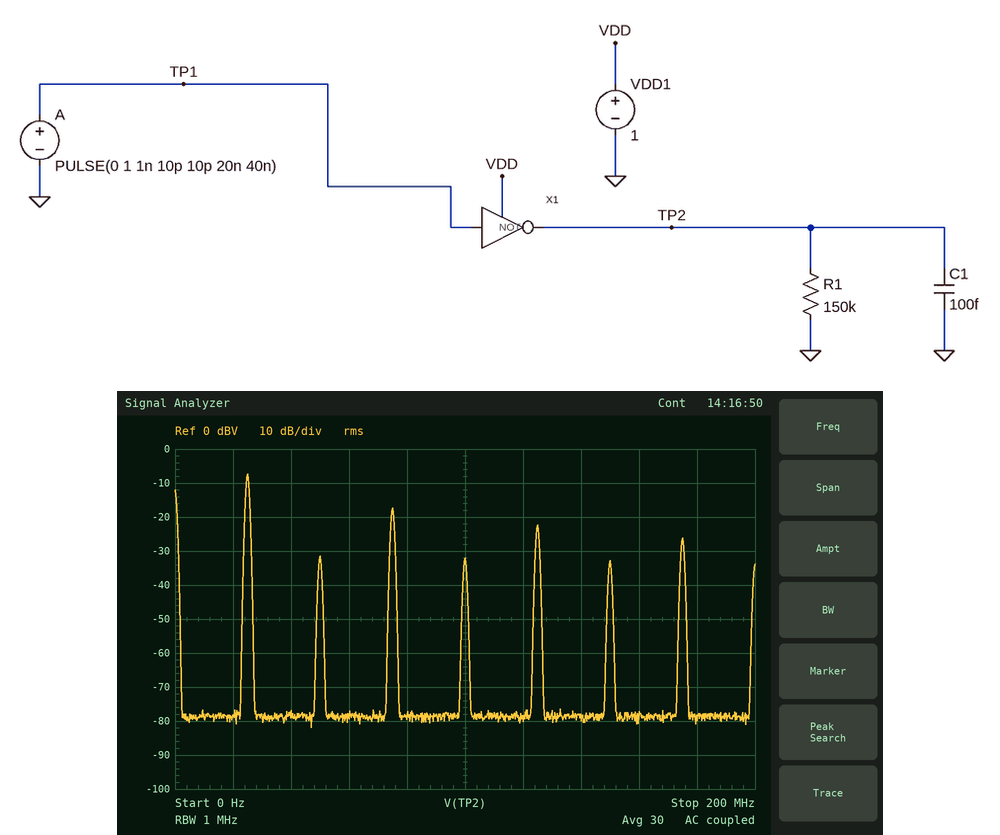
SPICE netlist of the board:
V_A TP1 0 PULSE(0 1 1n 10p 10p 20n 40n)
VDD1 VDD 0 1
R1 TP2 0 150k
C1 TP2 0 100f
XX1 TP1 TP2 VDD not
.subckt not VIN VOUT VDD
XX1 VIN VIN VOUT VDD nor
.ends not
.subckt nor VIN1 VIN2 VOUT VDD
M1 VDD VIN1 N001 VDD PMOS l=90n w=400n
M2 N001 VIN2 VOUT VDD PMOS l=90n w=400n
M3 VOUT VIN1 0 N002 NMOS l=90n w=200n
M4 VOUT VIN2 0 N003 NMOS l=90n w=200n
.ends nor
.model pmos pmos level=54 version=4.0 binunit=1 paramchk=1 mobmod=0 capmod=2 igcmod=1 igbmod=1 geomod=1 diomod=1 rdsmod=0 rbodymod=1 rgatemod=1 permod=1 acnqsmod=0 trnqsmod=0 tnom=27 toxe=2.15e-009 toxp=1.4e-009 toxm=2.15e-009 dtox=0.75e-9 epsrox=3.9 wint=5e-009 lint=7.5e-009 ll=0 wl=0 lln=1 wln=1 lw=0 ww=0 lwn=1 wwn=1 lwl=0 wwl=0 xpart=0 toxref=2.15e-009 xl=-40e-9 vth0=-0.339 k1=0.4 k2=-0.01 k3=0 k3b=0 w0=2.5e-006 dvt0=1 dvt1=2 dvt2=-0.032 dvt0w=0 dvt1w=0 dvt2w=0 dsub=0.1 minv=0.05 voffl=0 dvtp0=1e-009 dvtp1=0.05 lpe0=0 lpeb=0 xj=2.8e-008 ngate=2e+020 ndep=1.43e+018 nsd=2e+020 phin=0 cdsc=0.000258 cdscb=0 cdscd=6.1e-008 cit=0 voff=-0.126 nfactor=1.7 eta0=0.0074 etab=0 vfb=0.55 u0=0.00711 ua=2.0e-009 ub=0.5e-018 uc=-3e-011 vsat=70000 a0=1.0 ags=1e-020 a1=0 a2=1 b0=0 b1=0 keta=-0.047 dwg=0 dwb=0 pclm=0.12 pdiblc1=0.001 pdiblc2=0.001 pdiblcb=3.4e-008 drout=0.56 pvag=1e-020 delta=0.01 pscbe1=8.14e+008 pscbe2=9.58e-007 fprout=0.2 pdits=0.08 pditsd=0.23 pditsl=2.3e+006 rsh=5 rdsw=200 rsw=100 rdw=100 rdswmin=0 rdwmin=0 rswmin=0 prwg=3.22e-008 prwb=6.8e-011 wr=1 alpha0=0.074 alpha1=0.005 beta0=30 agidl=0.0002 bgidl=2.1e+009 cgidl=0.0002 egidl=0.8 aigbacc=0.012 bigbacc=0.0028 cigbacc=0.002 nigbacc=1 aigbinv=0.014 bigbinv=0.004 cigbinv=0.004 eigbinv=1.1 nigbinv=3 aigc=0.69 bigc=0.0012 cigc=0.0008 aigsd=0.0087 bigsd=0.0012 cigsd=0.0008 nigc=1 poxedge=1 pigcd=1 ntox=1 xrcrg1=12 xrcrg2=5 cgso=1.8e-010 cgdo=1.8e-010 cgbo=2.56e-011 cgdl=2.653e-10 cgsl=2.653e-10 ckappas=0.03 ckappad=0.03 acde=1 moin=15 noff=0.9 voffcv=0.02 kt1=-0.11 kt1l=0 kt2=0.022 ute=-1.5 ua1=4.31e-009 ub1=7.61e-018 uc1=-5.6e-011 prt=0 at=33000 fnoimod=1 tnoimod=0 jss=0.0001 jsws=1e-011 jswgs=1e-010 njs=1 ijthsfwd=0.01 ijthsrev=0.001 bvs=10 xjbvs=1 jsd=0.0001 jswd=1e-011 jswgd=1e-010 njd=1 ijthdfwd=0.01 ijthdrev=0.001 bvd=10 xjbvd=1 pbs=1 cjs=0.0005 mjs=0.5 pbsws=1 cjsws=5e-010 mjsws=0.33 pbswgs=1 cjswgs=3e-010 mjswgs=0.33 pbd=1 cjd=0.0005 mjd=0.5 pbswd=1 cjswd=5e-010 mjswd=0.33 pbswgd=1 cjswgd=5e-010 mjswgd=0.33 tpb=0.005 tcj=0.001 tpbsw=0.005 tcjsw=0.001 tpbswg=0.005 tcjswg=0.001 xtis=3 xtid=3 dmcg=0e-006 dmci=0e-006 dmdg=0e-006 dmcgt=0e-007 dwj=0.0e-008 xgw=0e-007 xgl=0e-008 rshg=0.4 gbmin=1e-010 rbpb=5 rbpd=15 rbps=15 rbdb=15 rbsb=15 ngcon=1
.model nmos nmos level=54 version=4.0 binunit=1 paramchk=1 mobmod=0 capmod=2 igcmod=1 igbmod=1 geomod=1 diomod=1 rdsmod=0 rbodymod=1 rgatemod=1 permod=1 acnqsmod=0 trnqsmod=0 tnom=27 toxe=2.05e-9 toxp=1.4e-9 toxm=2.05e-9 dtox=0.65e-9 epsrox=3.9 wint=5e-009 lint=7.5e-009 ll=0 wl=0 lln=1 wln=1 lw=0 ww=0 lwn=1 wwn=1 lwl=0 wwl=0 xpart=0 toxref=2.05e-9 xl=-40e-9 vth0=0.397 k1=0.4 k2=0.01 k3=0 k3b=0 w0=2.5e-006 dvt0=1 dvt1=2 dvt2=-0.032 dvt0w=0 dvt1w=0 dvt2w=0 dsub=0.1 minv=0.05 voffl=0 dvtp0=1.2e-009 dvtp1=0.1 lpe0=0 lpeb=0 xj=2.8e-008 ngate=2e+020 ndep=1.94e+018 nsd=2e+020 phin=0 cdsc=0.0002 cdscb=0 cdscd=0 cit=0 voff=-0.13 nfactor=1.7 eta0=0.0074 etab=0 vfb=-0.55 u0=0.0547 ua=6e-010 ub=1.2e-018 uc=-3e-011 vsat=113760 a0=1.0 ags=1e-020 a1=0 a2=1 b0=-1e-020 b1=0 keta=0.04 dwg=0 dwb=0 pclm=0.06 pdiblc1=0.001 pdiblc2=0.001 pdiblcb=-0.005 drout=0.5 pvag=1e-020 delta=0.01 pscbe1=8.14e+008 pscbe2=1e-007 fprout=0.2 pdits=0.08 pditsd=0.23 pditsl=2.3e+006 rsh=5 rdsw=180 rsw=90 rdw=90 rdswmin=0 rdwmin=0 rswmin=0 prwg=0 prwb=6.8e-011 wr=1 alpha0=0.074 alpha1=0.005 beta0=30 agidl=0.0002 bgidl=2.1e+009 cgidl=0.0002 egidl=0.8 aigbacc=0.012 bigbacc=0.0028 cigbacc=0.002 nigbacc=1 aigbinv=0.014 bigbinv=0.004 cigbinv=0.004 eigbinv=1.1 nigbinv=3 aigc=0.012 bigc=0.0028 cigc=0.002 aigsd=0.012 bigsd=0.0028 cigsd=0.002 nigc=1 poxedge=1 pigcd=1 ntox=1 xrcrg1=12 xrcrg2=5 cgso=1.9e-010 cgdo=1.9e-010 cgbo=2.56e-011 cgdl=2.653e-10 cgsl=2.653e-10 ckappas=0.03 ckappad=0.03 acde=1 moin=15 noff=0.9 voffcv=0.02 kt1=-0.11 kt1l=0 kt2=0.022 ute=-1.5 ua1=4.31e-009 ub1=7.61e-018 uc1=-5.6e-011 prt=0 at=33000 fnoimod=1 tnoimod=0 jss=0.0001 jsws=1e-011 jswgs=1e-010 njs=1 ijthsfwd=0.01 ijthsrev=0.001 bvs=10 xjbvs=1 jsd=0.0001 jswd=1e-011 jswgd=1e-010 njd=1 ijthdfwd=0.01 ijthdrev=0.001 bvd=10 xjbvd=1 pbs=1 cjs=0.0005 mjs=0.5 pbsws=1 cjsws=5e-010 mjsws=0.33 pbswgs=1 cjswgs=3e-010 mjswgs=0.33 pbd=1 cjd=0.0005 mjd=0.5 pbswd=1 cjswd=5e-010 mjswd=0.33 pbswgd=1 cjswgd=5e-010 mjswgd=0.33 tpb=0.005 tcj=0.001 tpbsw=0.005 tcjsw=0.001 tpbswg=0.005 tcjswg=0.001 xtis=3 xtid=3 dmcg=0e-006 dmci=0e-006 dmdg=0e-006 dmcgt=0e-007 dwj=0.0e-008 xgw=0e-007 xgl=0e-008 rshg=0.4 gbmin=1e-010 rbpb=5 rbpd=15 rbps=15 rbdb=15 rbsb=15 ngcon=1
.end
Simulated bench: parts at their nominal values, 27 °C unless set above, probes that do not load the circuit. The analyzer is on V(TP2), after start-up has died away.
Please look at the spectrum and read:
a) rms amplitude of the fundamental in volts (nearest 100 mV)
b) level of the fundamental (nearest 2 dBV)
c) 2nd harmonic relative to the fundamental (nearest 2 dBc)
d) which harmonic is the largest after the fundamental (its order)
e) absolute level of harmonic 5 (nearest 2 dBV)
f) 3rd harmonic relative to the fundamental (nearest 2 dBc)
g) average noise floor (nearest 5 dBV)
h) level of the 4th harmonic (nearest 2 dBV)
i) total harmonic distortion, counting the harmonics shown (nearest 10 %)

400 mV
-8 dBV
-24 dBc
3
-22 dBV
-10 dBc
-80 dBV
-32 dBV
40 %
